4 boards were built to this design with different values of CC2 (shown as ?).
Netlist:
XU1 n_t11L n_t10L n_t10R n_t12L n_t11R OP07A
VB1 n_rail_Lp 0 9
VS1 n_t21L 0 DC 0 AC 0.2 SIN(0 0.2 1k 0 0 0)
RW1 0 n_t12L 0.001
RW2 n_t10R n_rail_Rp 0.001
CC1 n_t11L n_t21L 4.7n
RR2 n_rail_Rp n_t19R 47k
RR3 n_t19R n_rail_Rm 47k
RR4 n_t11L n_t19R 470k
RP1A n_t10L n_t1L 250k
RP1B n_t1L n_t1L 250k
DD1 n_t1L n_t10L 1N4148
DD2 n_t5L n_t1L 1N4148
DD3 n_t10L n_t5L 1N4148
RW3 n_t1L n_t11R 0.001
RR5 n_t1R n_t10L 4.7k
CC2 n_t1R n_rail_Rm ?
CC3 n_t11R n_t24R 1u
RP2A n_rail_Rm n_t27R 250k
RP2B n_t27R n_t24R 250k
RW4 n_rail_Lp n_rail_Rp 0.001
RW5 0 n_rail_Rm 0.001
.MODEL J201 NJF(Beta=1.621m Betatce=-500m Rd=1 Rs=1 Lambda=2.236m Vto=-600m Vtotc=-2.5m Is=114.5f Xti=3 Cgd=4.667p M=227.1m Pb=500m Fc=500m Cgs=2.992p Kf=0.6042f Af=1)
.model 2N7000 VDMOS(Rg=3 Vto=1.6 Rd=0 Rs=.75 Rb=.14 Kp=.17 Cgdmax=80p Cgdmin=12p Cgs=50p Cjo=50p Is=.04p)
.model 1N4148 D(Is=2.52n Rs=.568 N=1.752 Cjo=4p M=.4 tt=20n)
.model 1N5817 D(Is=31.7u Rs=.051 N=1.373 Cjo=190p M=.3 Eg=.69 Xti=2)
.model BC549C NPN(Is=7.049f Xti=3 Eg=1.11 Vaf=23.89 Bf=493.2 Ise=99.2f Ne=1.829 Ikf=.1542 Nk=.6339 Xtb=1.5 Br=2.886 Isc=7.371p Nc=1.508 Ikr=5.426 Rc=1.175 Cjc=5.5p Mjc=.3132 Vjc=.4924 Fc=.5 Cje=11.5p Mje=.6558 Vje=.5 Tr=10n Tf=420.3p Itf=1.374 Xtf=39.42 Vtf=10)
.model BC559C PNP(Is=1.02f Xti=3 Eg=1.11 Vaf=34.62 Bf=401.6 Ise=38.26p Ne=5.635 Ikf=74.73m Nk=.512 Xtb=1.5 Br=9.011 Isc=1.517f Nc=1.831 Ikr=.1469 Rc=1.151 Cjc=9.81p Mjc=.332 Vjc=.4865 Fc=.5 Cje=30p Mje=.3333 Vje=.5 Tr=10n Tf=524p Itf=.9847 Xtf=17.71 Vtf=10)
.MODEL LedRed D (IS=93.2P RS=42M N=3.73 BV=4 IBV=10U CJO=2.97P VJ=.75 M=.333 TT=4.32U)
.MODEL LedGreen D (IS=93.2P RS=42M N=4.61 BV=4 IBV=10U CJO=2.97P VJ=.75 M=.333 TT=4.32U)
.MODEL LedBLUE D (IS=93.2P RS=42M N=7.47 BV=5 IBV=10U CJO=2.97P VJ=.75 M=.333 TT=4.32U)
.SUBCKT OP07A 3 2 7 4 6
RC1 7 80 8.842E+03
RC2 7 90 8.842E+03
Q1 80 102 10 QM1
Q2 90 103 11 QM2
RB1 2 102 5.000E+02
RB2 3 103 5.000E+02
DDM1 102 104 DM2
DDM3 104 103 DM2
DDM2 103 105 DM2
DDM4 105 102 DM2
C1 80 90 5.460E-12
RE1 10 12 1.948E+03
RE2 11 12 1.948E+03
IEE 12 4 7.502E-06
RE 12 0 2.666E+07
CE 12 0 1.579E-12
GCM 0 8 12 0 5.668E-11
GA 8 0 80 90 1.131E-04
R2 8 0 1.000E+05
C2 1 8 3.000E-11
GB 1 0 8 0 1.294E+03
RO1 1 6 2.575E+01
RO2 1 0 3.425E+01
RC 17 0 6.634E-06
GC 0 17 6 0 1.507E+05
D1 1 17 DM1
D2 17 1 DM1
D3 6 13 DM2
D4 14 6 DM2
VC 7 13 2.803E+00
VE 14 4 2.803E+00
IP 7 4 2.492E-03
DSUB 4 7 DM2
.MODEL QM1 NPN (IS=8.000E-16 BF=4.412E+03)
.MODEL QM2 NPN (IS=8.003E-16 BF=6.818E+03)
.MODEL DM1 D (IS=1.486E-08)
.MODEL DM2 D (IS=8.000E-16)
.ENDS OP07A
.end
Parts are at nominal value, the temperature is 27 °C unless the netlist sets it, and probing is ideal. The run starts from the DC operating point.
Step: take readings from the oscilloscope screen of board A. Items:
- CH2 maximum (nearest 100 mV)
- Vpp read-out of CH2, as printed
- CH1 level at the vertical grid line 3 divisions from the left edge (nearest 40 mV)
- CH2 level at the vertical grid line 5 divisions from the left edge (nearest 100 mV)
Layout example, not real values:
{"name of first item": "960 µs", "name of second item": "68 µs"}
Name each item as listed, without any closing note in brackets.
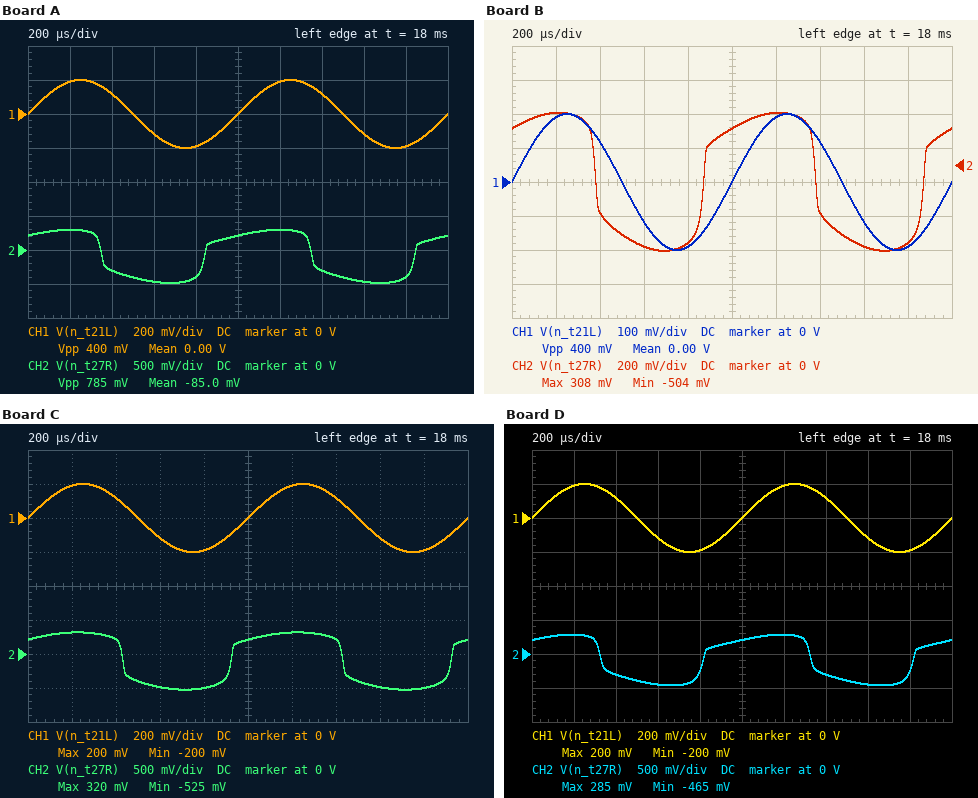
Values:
{"CH2 maximum": "300 mV", "Vpp read-out of CH2, as printed": "785 mV", "CH1 level at the vertical grid line 3 divisions from the left edge": "-120 mV", "CH2 level at the vertical grid line 5 divisions from the left edge": "200 mV"}
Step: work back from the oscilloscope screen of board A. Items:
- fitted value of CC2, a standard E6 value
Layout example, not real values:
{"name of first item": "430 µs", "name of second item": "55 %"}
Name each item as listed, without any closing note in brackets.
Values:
{"fitted value of CC2, a standard E6 value": "22 nF"}
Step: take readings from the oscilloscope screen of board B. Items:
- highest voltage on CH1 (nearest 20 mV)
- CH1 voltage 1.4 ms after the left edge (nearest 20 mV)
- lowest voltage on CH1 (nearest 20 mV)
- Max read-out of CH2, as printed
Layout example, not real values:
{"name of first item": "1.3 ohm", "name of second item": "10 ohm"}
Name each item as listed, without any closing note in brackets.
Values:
{"highest voltage on CH1": "200 mV", "CH1 voltage 1.4 ms after the left edge": "120 mV", "lowest voltage on CH1": "-200 mV", "Max read-out of CH2, as printed": "308 mV"}
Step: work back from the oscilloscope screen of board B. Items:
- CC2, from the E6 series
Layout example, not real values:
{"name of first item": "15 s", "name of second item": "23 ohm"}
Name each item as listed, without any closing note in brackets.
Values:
{"CC2, from the E6 series": "33 nF"}
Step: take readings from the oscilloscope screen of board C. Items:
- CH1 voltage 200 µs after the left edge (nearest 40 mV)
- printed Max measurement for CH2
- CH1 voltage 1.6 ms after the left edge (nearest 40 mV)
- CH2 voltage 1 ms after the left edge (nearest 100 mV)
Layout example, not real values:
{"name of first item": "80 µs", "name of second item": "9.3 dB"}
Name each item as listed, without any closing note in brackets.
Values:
{"CH1 voltage 200 µs after the left edge": "200 mV", "printed Max measurement for CH2": "320 mV", "CH1 voltage 1.6 ms after the left edge": "-120 mV", "CH2 voltage 1 ms after the left edge": "200 mV"}
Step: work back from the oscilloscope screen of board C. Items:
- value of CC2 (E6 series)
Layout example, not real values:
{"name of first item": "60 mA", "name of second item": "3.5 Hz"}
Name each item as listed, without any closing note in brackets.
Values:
{"value of CC2": "68 nF"}
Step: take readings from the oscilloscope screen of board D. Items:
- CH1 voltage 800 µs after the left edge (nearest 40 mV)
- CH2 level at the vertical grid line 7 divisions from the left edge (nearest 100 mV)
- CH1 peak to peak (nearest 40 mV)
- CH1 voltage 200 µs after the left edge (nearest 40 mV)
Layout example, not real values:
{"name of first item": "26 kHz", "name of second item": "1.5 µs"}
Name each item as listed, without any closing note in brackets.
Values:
{"CH1 voltage 800 µs after the left edge": "-200 mV", "CH2 level at the vertical grid line 7 divisions from the left edge": "-300 mV", "CH1 peak to peak": "400 mV", "CH1 voltage 200 µs after the left edge": "200 mV"}
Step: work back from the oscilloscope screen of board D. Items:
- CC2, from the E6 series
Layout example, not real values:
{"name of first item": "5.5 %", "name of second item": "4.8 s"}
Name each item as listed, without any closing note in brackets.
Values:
{"CC2, from the E6 series": "15 nF"}
